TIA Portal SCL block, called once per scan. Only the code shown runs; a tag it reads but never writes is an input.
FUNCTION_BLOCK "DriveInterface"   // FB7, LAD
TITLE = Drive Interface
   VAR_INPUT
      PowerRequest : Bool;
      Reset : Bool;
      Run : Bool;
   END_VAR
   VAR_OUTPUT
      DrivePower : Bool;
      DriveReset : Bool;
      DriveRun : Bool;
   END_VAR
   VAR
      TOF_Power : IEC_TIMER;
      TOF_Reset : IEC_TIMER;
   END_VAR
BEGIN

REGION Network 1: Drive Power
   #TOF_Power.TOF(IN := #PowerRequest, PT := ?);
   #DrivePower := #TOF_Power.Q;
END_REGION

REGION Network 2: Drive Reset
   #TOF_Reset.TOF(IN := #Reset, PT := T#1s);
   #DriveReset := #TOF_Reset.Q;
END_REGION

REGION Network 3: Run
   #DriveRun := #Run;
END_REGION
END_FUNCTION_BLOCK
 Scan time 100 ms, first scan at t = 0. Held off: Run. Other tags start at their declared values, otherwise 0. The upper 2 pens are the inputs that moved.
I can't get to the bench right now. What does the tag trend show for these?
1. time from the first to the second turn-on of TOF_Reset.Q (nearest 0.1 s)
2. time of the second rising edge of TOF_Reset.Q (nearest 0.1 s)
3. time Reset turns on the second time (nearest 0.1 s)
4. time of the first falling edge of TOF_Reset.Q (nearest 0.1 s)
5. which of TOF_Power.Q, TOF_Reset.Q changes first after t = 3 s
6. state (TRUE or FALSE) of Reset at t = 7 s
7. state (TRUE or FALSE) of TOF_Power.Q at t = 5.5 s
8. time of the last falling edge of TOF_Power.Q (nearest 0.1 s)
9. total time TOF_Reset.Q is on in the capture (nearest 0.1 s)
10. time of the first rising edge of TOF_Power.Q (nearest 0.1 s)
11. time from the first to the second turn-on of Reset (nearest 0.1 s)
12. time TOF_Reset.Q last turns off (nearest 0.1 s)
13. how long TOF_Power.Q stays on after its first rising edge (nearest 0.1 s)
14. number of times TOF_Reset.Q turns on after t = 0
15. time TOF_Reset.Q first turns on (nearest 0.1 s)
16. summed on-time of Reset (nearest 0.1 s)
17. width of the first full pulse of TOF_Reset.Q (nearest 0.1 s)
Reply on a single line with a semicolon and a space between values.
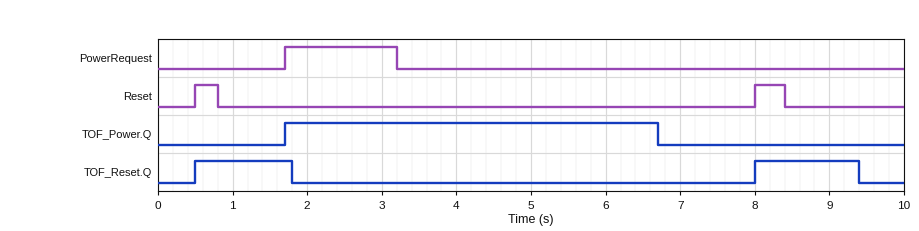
7.5 s; 8.0 s; 8.0 s; 1.8 s; TOF_Power.Q; FALSE; TRUE; 6.7 s; 2.7 s; 1.7 s; 7.5 s; 9.4 s; 5.0 s; 2; 0.5 s; 0.7 s; 1.3 s
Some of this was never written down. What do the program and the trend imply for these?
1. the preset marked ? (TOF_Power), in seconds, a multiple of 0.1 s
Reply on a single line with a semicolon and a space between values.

3.5 s
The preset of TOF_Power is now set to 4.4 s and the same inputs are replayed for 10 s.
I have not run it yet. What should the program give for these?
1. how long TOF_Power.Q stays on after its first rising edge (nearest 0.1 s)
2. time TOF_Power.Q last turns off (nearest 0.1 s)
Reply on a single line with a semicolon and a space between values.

5.9 s; 7.6 s
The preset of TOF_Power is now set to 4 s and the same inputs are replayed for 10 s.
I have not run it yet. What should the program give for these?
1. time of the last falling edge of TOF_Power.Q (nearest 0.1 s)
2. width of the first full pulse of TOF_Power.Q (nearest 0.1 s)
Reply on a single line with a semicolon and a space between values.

7.2 s; 5.5 s
